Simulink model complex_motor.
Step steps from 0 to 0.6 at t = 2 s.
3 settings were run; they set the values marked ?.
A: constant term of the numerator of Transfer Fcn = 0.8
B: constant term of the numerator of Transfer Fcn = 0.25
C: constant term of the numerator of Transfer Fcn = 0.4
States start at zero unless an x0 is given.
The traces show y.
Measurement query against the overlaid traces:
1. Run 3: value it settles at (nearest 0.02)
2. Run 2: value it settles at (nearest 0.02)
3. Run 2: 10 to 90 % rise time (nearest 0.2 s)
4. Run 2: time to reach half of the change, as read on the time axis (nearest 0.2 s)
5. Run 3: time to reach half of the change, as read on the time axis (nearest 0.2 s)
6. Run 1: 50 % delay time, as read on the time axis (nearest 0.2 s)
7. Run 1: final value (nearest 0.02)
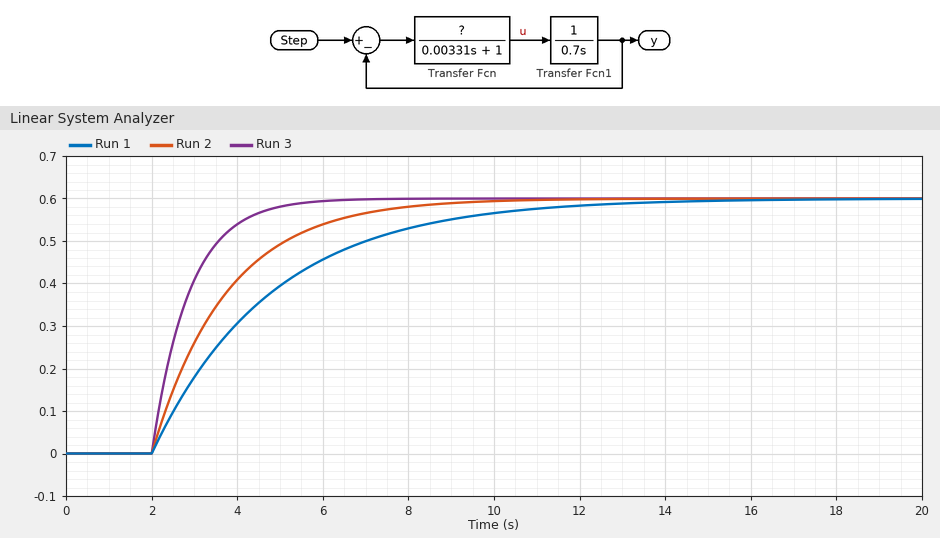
0.60
0.60
3.8 s
3.2 s
2.6 s
4.0 s
0.60
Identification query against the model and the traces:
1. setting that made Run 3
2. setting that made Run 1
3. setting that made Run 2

A
B
C
